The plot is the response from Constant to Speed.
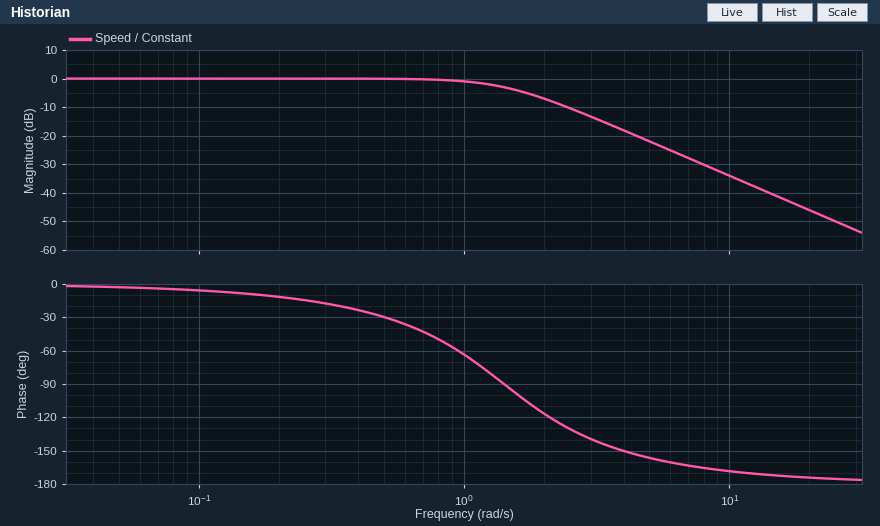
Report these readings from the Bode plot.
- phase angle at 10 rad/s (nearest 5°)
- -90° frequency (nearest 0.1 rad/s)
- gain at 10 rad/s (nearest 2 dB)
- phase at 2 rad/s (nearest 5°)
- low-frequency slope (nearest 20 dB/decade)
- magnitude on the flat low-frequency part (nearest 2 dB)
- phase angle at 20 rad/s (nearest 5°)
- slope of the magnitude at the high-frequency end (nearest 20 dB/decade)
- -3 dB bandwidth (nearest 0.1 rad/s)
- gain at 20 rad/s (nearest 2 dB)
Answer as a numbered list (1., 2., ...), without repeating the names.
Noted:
1. -170°
2. 1.4 rad/s
3. -34 dB
4. -115°
5. 0 dB/decade
6. 0 dB
7. -175°
8. -40 dB/decade
9. 1.4 rad/s
10. -46 dB
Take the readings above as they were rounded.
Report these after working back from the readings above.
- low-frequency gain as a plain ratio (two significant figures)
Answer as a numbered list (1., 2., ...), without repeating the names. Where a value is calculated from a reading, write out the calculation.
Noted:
1. 10^(0 / 20) = 1.0
